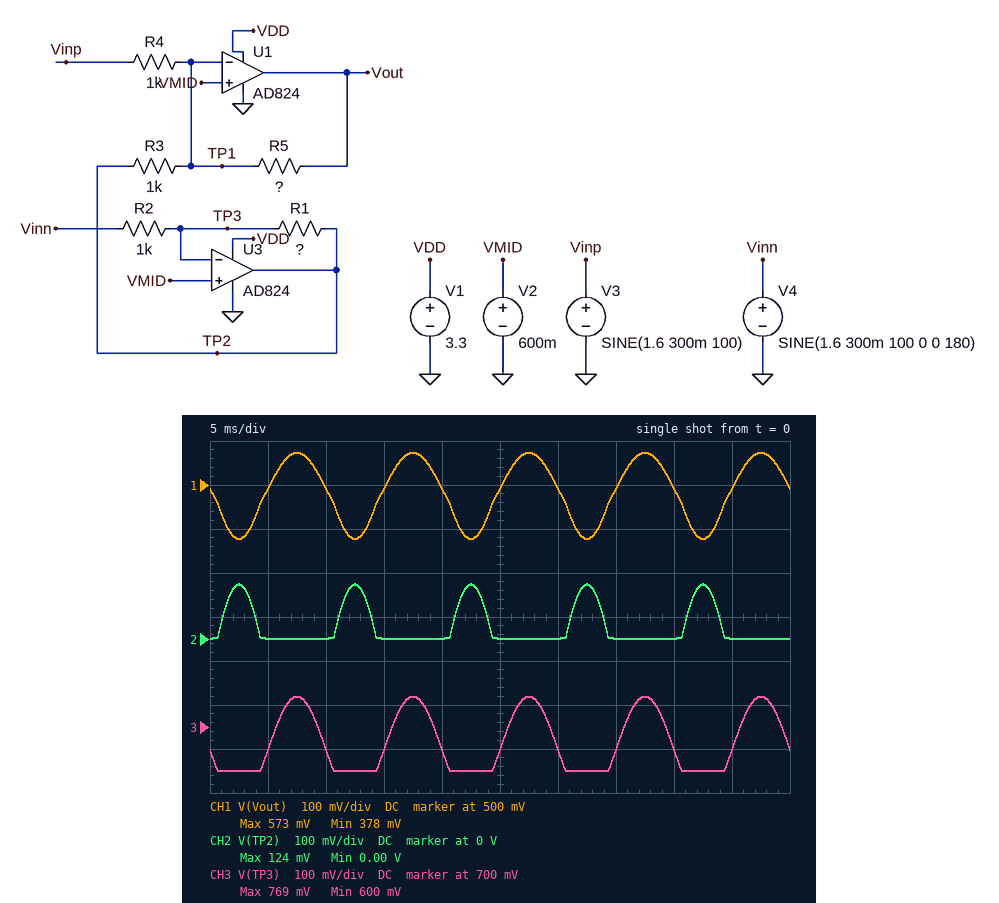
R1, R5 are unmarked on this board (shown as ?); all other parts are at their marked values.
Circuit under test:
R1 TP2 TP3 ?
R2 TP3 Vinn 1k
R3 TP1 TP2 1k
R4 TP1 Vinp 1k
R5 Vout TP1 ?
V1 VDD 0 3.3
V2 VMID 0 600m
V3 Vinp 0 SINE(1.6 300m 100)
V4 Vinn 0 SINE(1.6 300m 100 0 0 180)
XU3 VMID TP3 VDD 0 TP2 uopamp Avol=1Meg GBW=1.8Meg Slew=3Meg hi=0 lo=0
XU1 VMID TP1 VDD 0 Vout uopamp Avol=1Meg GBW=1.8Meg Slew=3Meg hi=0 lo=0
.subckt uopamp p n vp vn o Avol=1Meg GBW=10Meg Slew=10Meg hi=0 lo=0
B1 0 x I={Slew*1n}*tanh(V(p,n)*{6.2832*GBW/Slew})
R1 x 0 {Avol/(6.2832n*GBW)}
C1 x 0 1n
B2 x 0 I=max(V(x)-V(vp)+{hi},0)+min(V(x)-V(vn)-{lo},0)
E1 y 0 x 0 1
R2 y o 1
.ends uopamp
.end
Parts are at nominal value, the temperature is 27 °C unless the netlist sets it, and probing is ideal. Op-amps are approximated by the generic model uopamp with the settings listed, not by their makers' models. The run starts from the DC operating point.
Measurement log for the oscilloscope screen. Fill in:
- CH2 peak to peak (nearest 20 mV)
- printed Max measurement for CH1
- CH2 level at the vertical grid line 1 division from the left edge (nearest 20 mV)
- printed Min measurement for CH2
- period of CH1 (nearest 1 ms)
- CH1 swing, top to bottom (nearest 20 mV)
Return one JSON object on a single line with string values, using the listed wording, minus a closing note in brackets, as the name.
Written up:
{"CH2 peak to peak": "120 mV", "printed Max measurement for CH1": "573 mV", "CH2 level at the vertical grid line 1 division from the left edge": "0 V", "printed Min measurement for CH2": "0.00 V", "period of CH1": "10 ms", "CH1 swing, top to bottom": "200 mV"}
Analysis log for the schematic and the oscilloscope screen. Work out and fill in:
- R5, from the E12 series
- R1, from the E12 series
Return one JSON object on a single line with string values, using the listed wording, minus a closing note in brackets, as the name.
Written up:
{"R5, from the E12 series": "270 Ω", "R1, from the E12 series": "680 Ω"}
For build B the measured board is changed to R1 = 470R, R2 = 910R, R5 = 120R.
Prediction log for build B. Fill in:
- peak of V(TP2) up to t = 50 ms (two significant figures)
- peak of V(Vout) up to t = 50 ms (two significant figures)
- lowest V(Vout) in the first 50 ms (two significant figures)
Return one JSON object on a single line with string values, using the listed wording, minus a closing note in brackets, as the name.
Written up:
{"peak of V(TP2) up to t = 50 ms": "240 mV", "peak of V(Vout) up to t = 50 ms": "590 mV", "lowest V(Vout) in the first 50 ms": "490 mV"}
